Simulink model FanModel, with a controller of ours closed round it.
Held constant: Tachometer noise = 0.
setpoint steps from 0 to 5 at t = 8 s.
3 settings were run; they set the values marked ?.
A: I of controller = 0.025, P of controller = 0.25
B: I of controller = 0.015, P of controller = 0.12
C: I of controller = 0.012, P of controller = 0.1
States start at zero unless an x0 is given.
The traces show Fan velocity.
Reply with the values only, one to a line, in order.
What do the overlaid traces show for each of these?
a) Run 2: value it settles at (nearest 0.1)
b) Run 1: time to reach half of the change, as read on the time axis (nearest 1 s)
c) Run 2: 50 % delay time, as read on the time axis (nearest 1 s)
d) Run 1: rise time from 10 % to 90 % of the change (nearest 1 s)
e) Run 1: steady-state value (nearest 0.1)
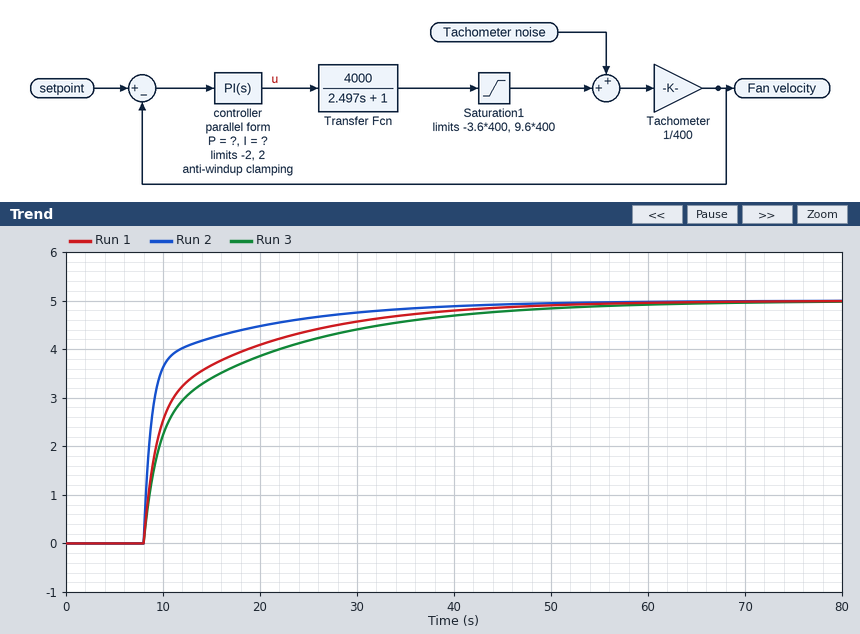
5.0
10 s
9 s
20 s
5.0
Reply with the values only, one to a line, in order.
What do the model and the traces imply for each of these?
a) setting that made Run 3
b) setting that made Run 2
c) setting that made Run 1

C
A
B
